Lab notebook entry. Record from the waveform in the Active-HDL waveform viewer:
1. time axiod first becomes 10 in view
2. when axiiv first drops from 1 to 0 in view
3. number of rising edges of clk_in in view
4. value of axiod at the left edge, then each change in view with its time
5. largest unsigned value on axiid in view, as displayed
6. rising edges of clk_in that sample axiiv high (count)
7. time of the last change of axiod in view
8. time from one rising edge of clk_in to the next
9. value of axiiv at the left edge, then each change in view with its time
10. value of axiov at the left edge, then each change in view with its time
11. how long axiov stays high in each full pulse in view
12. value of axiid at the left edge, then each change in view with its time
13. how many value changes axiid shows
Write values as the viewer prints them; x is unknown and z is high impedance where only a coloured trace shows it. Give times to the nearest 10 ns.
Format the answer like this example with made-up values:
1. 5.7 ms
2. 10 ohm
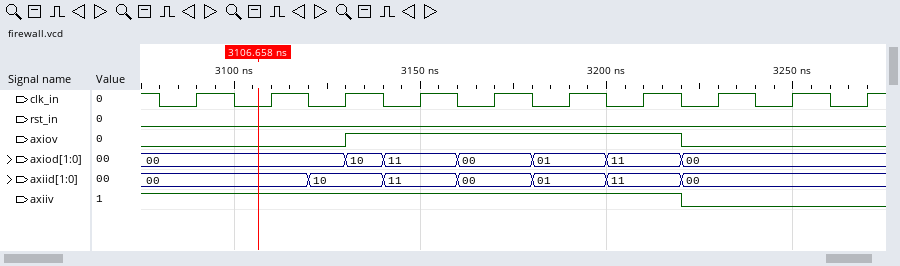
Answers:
1. 3130 ns
2. 3220 ns
3. 10
4. 00, 10 at 3130 ns, 11 at 3140 ns, 00 at 3160 ns, 01 at 3180 ns, 11 at 3200 ns, 00 at 3220 ns
5. 11
6. 7
7. 3220 ns
8. 20 ns
9. 1, 0 at 3220 ns
10. 0, 1 at 3130 ns, 0 at 3220 ns
11. 90 ns
12. 00, 10 at 3120 ns, 11 at 3140 ns, 00 at 3160 ns, 01 at 3180 ns, 11 at 3200 ns, 00 at 3220 ns
13. 6
